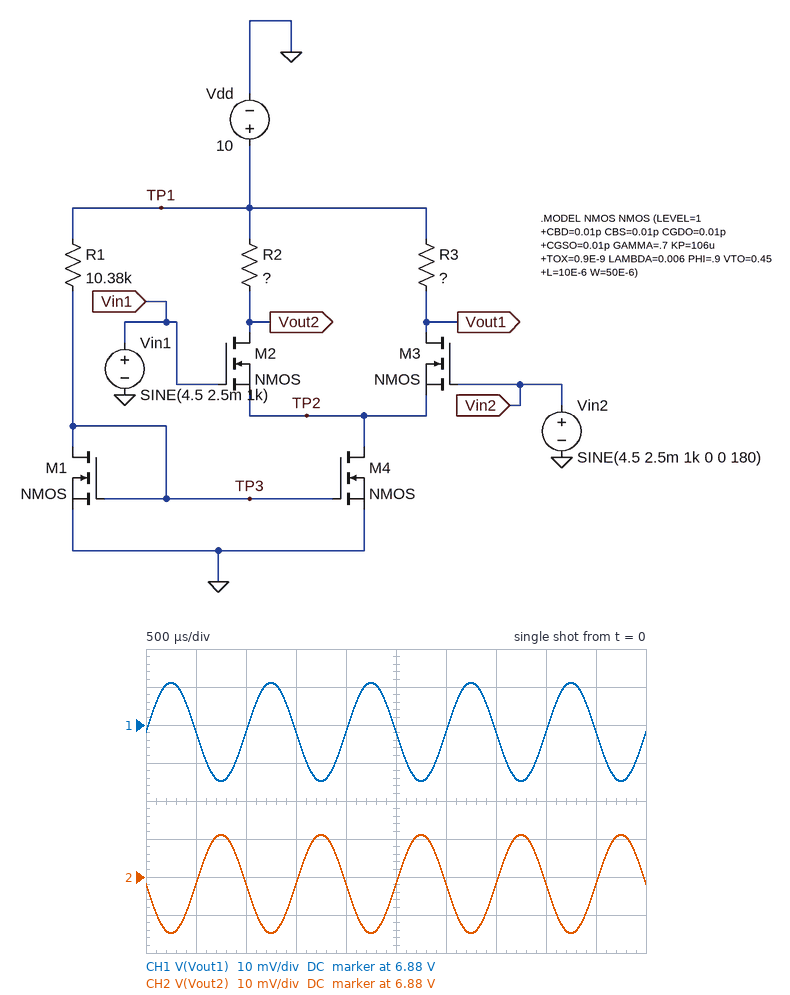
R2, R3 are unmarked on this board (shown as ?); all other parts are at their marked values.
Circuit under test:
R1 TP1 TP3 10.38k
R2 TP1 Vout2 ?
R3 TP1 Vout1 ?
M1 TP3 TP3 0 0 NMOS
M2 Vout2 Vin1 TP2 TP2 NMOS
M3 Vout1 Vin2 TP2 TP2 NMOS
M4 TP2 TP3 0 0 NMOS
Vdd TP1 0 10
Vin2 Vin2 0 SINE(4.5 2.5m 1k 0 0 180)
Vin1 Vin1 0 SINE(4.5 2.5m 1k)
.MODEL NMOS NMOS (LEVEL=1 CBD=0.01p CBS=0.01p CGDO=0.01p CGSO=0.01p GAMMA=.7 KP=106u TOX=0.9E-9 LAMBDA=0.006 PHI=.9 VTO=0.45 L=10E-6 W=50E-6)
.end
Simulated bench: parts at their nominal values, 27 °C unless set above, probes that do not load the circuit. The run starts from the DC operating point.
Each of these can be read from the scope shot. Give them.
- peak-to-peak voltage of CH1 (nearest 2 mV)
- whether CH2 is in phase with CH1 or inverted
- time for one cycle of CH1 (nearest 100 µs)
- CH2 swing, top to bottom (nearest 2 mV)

26 mV
inverted
1.0 ms
26 mV
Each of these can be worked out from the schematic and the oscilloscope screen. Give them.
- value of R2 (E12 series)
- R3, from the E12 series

8.2 kΩ
8.2 kΩ
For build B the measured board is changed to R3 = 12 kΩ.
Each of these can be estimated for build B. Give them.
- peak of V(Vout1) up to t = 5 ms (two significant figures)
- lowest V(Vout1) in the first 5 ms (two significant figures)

5.5 V
5.4 V
